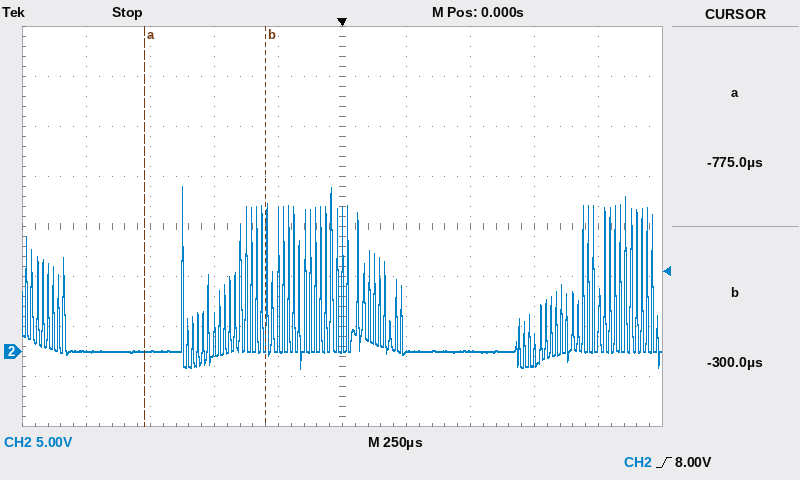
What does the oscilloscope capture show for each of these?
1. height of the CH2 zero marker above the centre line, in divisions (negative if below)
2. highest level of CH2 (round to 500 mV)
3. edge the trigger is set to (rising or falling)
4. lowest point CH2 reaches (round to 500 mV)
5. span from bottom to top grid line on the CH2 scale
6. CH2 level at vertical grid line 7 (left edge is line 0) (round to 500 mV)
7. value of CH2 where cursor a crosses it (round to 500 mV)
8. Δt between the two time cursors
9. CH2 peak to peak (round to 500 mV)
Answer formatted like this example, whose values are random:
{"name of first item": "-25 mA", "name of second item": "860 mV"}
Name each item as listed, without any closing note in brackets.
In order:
{"height of the CH2 zero marker above the centre line, in divisions": "-2.5 div", "highest level of CH2": "16.5 V", "edge the trigger is set to": "rising", "lowest point CH2 reaches": "-1.5 V", "span from bottom to top grid line on the CH2 scale": "40 V", "CH2 level at vertical grid line 7 (left edge is line 0)": "0.0 V", "value of CH2 where cursor a crosses it": "0.0 V", "Δt between the two time cursors": "475 µs", "CH2 peak to peak": "18.0 V"}
